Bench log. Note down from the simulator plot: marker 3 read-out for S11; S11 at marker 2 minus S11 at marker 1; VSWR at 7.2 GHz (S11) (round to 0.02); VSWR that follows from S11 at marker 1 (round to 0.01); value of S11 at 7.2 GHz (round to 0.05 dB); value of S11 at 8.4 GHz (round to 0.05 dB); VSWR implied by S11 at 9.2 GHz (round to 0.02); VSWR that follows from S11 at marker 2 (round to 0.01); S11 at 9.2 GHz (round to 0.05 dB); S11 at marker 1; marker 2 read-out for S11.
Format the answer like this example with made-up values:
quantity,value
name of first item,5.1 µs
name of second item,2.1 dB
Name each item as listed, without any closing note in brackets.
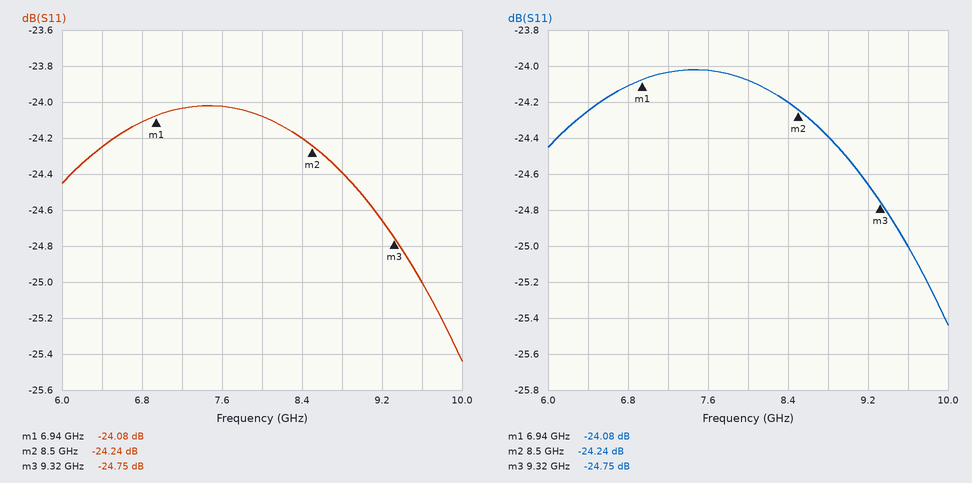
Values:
quantity,value
marker 3 read-out for S11,-24.75 dB
S11 at marker 2 minus S11 at marker 1,-0.16 dB
VSWR at 7.2 GHz (S11),1.14
VSWR that follows from S11 at marker 1,1.13
value of S11 at 7.2 GHz,-24.05 dB
value of S11 at 8.4 GHz,-24.20 dB
VSWR implied by S11 at 9.2 GHz,1.12
VSWR that follows from S11 at marker 2,1.13
S11 at 9.2 GHz,-24.65 dB
S11 at marker 1,-24.08 dB
marker 2 read-out for S11,-24.24 dB
